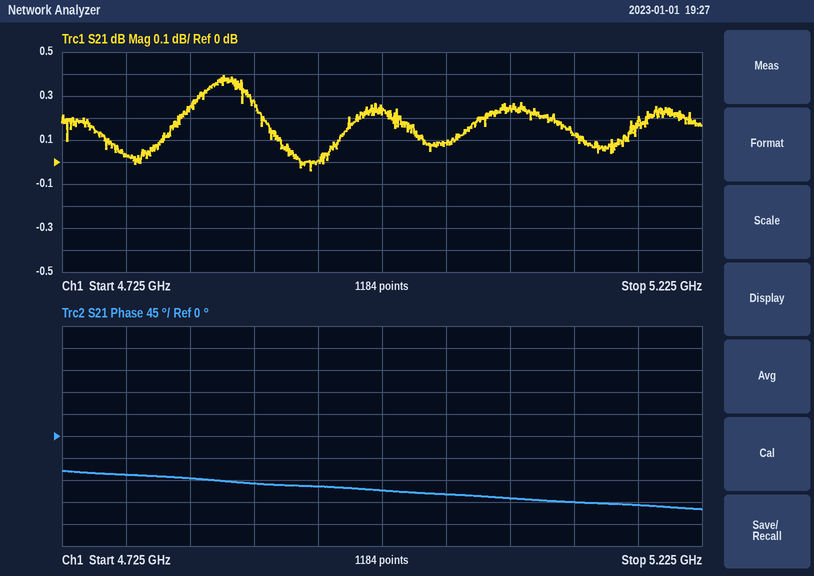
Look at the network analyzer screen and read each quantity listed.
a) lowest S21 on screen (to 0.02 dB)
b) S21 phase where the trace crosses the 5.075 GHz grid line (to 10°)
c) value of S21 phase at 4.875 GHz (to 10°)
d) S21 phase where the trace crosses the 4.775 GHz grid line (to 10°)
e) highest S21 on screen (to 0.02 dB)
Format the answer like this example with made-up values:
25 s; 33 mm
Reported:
-0.04 dB; -130°; -100°; -80°; 0.40 dB
